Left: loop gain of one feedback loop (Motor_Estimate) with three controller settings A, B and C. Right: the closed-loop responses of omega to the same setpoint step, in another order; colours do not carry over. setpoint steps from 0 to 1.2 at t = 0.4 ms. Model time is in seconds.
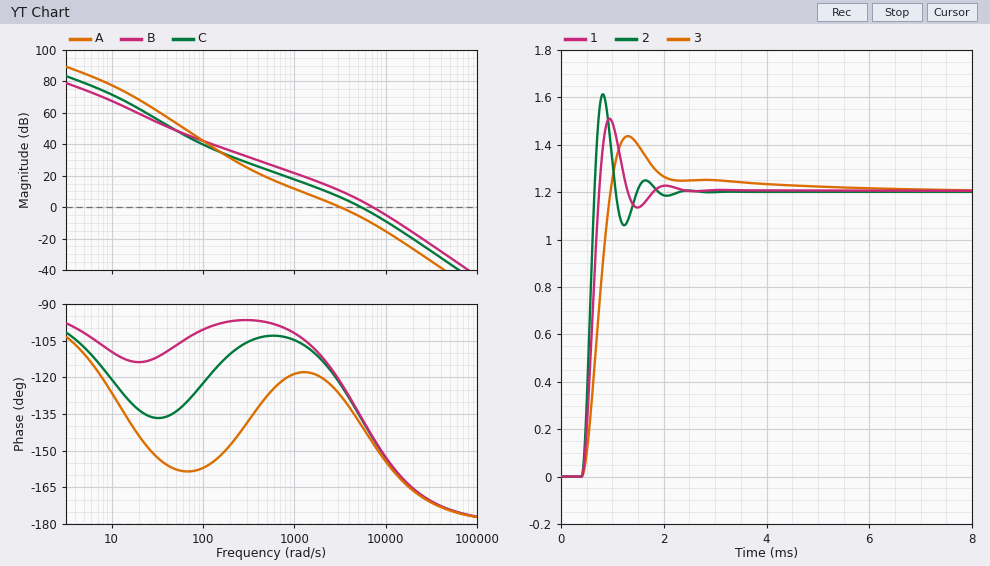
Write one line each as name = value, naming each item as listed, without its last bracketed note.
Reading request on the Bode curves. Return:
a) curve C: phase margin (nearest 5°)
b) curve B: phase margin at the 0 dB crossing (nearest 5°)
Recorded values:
curve C: phase margin = 45°
curve B: phase margin at the 0 dB crossing = 35°
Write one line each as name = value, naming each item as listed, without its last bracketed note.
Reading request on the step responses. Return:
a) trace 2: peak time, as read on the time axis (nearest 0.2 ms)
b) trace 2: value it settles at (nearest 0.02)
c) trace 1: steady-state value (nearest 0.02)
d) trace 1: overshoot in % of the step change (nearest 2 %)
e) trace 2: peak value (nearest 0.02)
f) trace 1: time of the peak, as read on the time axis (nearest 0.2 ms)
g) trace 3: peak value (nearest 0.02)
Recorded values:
trace 2: peak time, as read on the time axis = 0.8 ms
trace 2: value it settles at = 1.20
trace 1: steady-state value = 1.20
trace 1: overshoot in % of the step change = 26 %
trace 2: peak value = 1.62
trace 1: time of the peak, as read on the time axis = 1.0 ms
trace 3: peak value = 1.44
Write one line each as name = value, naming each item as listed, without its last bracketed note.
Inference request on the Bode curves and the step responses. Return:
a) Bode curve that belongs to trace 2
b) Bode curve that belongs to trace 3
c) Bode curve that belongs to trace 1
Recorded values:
Bode curve that belongs to trace 2 = B
Bode curve that belongs to trace 3 = A
Bode curve that belongs to trace 1 = C
